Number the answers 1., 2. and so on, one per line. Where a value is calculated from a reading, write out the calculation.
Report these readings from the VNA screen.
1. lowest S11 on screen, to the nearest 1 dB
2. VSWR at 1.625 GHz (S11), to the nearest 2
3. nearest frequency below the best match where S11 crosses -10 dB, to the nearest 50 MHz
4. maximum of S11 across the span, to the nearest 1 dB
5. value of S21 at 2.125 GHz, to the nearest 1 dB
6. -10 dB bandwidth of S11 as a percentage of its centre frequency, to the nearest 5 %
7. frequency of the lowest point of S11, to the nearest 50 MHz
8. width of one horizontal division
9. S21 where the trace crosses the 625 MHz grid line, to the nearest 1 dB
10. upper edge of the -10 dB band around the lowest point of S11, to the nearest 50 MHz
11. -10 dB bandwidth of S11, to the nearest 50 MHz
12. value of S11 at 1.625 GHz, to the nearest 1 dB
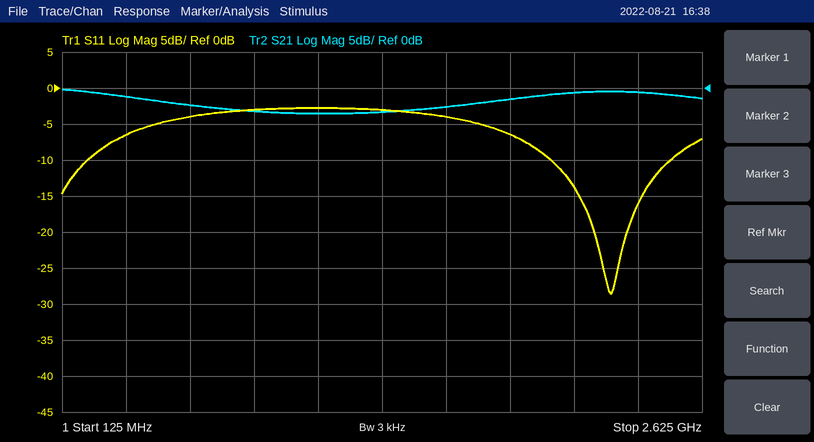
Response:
1. -29 dB
2. |Γ| = 10^(-4/20) = 0.6310; VSWR = (1 + 0.6310)/(1 − 0.6310) ≈ 4
3. 2.05 GHz
4. -3 dB
5. -1 dB
6. 450 MHz / 2.275 GHz ≈ 20 %
7. 2.25 GHz
8. 250 MHz
9. -2 dB
10. 2.50 GHz
11. 2.50 GHz − 2.05 GHz = 450 MHz
12. -4 dB
